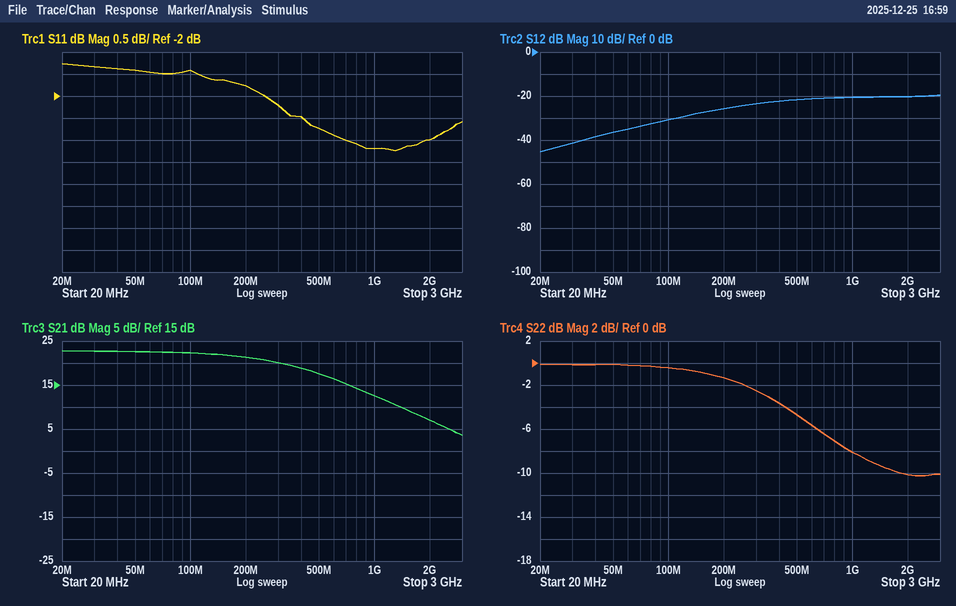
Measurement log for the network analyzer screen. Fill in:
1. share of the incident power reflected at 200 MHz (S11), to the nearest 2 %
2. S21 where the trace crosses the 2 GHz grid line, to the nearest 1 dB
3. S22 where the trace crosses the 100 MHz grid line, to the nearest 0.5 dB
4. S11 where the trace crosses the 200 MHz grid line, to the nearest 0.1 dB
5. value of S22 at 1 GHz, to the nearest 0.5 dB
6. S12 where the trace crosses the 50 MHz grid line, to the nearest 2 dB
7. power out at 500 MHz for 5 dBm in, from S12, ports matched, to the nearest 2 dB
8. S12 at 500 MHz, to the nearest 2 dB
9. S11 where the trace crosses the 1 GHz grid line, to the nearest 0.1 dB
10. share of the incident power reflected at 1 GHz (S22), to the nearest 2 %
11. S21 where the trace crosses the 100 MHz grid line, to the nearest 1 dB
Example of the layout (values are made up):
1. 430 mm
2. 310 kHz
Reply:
1. 66 %
2. 7 dB
3. -0.5 dB
4. -1.8 dB
5. -8.0 dB
6. -36 dB
7. -16 dBm
8. -22 dB
9. -3.2 dB
10. 16 %
11. 22 dB
